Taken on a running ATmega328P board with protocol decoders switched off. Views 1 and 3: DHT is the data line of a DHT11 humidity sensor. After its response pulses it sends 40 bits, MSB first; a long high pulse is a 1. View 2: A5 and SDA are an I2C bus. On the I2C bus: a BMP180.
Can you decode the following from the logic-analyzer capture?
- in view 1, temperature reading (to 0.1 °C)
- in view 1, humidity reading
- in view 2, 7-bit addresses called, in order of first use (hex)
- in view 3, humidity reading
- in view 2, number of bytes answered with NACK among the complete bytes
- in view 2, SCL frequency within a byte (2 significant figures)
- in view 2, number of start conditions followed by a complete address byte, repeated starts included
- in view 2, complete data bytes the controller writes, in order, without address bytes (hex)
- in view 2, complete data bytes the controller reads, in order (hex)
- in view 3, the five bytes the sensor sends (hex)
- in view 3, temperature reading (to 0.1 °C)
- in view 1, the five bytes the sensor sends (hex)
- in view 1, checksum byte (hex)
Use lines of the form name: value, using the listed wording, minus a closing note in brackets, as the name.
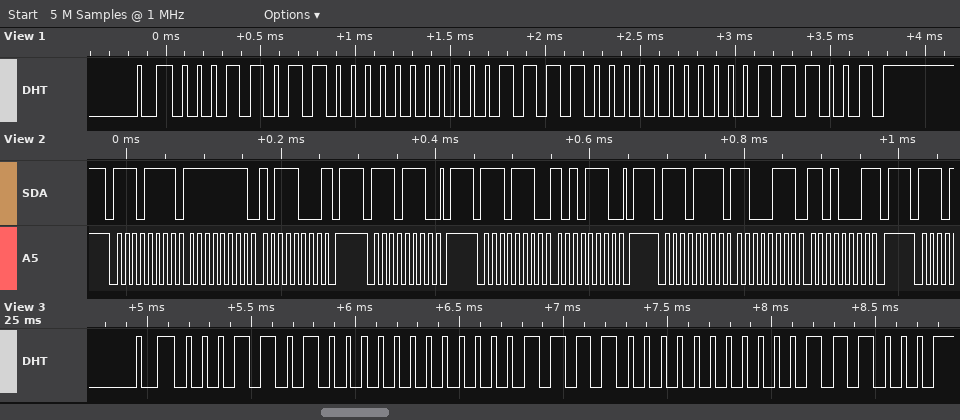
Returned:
in view 1, temperature reading: 30.0 °C
in view 1, humidity reading: 27 %
in view 2, 7-bit addresses called, in order of first use: 0x77
in view 3, humidity reading: 26 %
in view 2, number of bytes answered with NACK among the complete bytes: 2
in view 2, SCL frequency within a byte: 100 kHz
in view 2, number of start conditions followed by a complete address byte, repeated starts included: 4
in view 2, complete data bytes the controller writes, in order, without address bytes: AE
in view 2, complete data bytes the controller reads, in order: FF B8 C7 D1
in view 3, the five bytes the sensor sends: 1A 00 1E 00 38
in view 3, temperature reading: 30.0 °C
in view 1, the five bytes the sensor sends: 1B 00 1E 00 39
in view 1, checksum byte: 0x39
